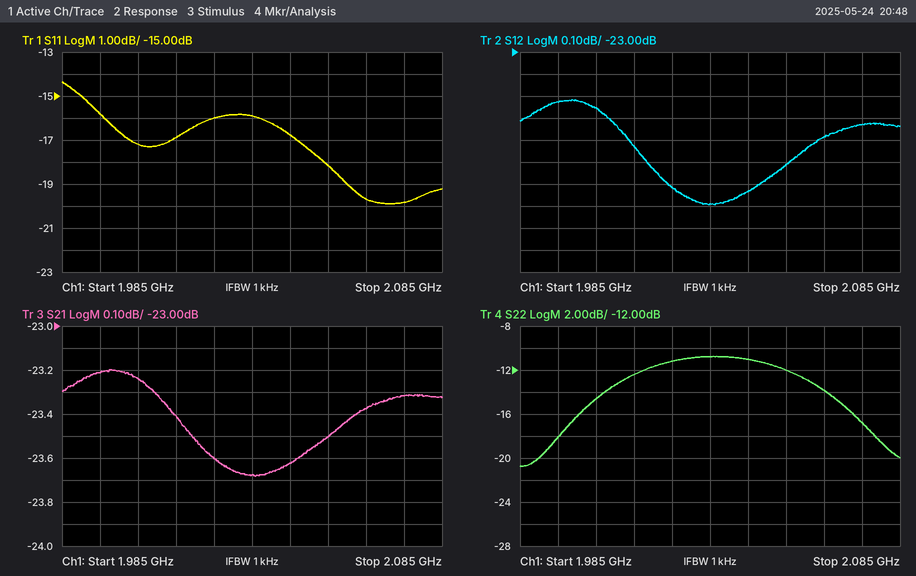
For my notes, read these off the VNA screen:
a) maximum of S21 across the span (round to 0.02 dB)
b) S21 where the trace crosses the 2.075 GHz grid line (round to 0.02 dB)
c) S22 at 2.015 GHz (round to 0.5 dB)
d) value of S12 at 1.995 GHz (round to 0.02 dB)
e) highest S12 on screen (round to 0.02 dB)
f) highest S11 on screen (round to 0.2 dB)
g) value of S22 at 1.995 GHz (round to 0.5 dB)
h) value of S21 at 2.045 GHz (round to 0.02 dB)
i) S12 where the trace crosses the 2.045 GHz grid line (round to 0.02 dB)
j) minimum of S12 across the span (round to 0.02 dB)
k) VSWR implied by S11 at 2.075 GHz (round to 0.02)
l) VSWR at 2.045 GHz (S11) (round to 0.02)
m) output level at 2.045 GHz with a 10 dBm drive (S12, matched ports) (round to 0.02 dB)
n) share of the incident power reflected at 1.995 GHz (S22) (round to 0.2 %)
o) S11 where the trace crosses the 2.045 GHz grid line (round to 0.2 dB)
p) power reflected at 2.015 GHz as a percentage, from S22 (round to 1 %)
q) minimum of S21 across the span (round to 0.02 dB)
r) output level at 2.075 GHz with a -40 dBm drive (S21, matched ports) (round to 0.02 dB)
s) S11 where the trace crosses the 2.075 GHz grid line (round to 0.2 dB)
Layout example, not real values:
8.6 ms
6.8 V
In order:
-23.20 dB
-23.32 dB
-12.5 dB
-23.22 dB
-23.22 dB
-14.4 dB
-18.0 dB
-23.62 dB
-23.64 dB
-23.70 dB
1.22
1.34
-13.64 dBm
1.6 %
-16.8 dB
6 %
-23.68 dB
-63.32 dBm
-19.8 dB
